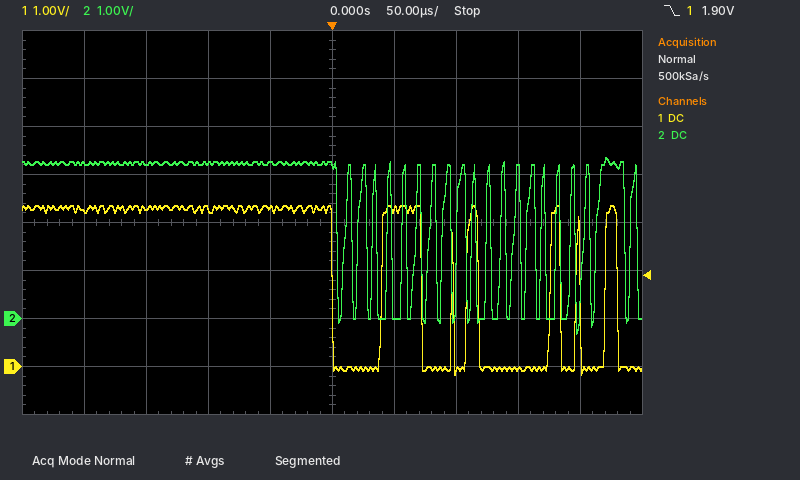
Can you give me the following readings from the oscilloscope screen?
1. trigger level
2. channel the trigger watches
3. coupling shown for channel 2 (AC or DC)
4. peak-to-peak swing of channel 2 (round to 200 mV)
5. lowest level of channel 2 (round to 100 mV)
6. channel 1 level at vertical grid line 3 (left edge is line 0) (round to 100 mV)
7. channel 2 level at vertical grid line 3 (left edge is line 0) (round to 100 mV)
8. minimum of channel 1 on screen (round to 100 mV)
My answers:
1.90 V
channel 1
DC
3.6 V
-300 mV
3.3 V
3.2 V
-200 mV
